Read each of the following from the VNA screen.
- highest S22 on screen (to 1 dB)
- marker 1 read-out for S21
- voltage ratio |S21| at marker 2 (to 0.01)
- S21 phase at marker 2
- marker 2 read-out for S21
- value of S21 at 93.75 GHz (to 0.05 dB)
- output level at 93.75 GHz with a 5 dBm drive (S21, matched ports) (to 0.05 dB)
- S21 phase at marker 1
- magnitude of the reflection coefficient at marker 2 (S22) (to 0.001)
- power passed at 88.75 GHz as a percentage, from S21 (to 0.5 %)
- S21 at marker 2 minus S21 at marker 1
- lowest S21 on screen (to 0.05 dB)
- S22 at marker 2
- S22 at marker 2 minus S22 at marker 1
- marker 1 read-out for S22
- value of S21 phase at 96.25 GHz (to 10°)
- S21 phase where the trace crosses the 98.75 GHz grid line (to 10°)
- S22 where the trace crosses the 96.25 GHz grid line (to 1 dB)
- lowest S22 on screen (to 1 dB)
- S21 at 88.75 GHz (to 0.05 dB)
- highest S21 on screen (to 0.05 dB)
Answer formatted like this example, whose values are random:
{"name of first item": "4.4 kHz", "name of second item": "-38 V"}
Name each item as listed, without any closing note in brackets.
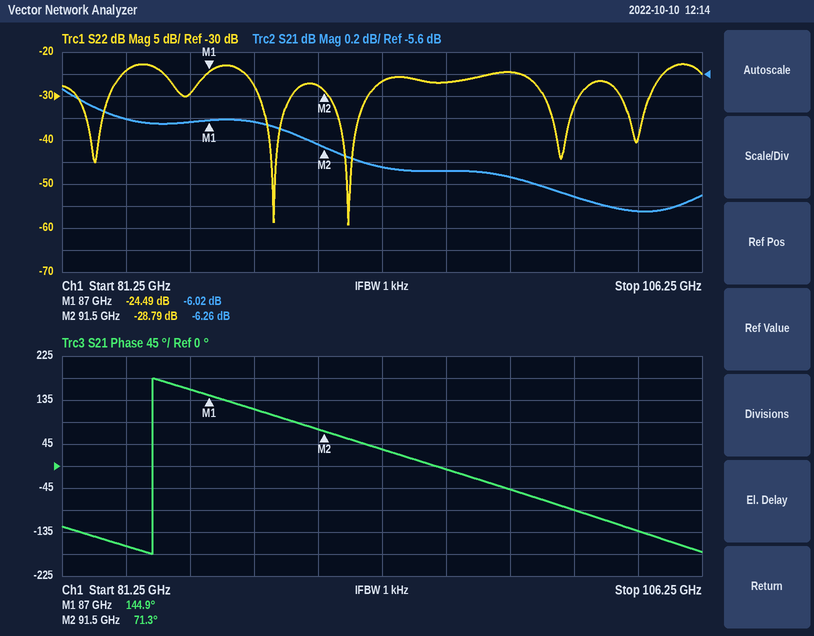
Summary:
{"highest S22 on screen": "-23 dB", "marker 1 read-out for S21": "-6.02 dB", "voltage ratio |S21| at marker 2": "0.49", "S21 phase at marker 2": "71.3°", "marker 2 read-out for S21": "-6.26 dB", "value of S21 at 93.75 GHz": "-6.45 dB", "output level at 93.75 GHz with a 5 dBm drive (S21, matched ports)": "-1.45 dBm", "S21 phase at marker 1": "144.9°", "magnitude of the reflection coefficient at marker 2 (S22)": "0.036", "power passed at 88.75 GHz as a percentage, from S21": "25.0 %", "S21 at marker 2 minus S21 at marker 1": "-0.24 dB", "lowest S21 on screen": "-6.85 dB", "S22 at marker 2": "-28.79 dB", "S22 at marker 2 minus S22 at marker 1": "-4.30 dB", "marker 1 read-out for S22": "-24.49 dB", "value of S21 phase at 96.25 GHz": "-10°", "S21 phase where the trace crosses the 98.75 GHz grid line": "-50°", "S22 where the trace crosses the 96.25 GHz grid line": "-27 dB", "lowest S22 on screen": "-59 dB", "S21 at 88.75 GHz": "-6.05 dB", "highest S21 on screen": "-5.75 dB"}
